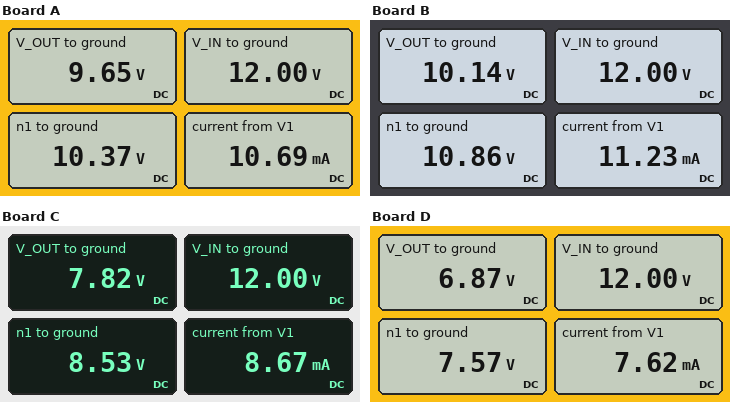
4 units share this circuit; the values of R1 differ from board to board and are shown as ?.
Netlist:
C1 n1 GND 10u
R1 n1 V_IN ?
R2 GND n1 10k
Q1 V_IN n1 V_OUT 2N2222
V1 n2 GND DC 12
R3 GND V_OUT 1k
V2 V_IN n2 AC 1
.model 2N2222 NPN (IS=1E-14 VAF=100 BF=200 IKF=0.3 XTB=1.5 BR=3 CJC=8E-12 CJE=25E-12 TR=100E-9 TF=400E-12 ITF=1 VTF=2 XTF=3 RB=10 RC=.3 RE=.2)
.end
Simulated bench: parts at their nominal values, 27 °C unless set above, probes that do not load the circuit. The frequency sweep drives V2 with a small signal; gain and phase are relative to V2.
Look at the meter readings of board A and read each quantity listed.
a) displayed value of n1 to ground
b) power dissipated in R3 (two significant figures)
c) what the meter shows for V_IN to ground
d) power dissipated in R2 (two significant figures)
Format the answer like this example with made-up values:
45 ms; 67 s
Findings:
10.37 V; 93 mW; 12.00 V; 11 mW
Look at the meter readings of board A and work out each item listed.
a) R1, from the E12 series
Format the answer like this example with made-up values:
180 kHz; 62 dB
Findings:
1.5 kΩ
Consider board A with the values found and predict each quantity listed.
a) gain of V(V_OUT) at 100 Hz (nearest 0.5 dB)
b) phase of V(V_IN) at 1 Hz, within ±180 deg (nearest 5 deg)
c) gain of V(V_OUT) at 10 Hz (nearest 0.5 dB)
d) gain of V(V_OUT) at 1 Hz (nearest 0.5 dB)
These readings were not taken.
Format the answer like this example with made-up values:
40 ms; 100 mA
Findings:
-19.5 dB; 0 deg; -3.5 dB; -1.5 dB
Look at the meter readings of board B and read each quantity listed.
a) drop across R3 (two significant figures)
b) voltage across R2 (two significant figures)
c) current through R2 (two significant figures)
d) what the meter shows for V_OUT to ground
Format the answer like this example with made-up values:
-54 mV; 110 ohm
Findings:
10 V; 11 V; 1.1 mA; 10.14 V
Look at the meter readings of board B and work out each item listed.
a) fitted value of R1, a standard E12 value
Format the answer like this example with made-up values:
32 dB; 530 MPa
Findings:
1 kΩ
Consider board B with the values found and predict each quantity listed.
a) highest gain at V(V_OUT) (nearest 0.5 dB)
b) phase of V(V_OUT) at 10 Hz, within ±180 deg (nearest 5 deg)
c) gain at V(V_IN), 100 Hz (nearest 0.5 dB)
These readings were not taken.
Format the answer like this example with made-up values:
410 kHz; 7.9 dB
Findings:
-1.0 dB; -30 deg; 0 dB
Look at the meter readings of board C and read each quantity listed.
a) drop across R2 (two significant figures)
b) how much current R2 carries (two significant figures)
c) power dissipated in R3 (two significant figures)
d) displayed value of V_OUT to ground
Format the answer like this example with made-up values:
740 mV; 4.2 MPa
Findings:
8.5 V; 850 µA; 61 mW; 7.82 V
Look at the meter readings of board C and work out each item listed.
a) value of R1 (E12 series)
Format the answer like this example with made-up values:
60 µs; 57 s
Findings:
3.9 kΩ
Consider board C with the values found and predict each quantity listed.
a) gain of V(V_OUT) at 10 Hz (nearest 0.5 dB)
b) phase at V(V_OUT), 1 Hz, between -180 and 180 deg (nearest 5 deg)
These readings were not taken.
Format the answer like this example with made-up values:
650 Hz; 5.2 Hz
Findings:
-9.0 dB; -10 deg
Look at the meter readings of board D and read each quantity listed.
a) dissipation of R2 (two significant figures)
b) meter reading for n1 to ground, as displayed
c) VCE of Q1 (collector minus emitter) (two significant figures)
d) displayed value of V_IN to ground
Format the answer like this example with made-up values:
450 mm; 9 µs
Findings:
5.7 mW; 7.57 V; 5.1 V; 12.00 V
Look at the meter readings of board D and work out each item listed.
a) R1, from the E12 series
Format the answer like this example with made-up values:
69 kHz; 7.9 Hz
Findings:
5.6 kΩ
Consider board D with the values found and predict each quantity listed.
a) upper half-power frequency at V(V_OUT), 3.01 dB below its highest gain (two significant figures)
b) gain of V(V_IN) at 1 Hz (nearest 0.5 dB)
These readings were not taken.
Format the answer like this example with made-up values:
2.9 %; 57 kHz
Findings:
4.5 Hz; 0 dB
